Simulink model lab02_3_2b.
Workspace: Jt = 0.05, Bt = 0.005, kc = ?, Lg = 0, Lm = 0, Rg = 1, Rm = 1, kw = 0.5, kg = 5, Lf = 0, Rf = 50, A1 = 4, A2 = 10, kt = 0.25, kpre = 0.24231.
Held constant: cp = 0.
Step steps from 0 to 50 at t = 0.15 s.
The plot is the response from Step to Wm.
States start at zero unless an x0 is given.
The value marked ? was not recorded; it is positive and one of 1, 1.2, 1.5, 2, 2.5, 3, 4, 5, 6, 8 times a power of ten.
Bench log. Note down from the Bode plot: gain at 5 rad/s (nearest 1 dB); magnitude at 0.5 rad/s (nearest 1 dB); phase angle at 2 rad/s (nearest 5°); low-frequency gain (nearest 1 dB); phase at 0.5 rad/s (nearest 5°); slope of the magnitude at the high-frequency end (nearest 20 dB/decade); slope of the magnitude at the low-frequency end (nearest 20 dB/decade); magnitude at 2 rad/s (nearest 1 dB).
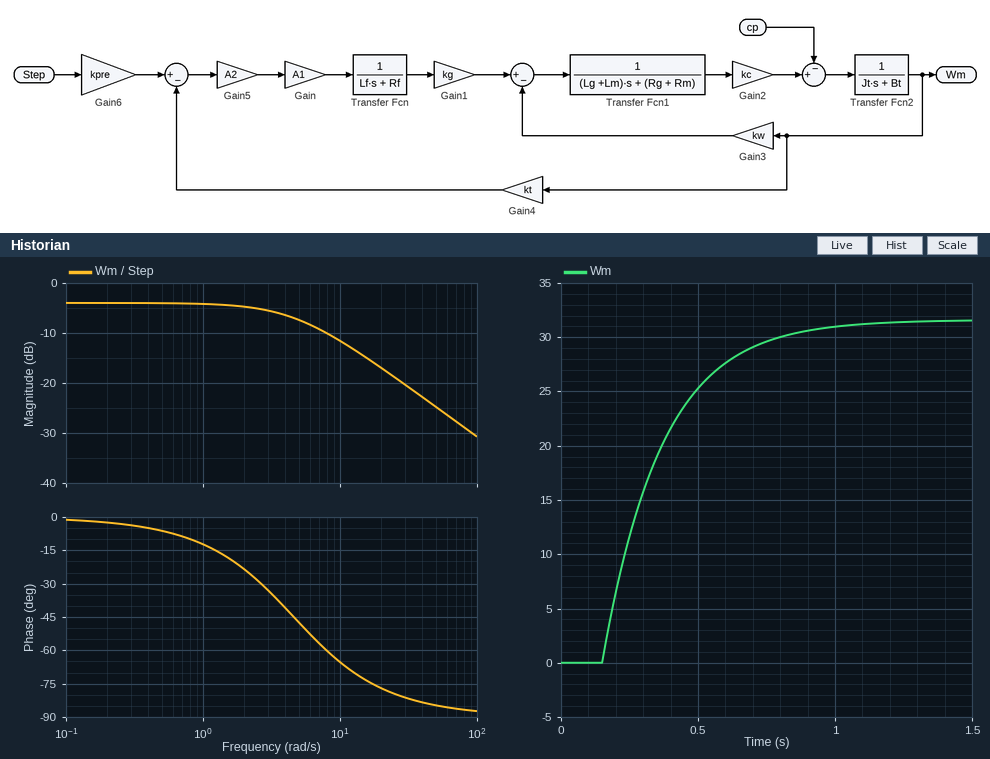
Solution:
-7 dB
-4 dB
-25°
-4 dB
-5°
-20 dB/decade
0 dB/decade
-5 dB
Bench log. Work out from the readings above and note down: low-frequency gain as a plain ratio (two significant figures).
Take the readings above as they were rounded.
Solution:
0.63
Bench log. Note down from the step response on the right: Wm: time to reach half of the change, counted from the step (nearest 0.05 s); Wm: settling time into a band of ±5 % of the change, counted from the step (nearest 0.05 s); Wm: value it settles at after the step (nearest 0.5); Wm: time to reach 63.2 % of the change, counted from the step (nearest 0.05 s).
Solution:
0.15 s
0.65 s
31.5
0.20 s
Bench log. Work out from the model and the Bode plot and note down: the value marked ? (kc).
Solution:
0.3
